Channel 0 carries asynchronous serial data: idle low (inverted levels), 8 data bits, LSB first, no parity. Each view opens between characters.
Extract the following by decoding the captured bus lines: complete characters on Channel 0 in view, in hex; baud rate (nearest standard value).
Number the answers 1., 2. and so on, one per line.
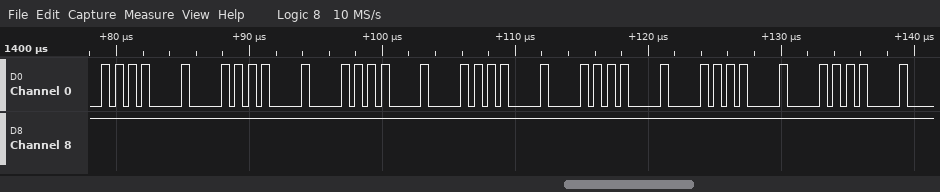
1. D5, 5F, 7D, D5, 5F, 7D, D5, 5F, 7D, D5
2. 2000000 baud
